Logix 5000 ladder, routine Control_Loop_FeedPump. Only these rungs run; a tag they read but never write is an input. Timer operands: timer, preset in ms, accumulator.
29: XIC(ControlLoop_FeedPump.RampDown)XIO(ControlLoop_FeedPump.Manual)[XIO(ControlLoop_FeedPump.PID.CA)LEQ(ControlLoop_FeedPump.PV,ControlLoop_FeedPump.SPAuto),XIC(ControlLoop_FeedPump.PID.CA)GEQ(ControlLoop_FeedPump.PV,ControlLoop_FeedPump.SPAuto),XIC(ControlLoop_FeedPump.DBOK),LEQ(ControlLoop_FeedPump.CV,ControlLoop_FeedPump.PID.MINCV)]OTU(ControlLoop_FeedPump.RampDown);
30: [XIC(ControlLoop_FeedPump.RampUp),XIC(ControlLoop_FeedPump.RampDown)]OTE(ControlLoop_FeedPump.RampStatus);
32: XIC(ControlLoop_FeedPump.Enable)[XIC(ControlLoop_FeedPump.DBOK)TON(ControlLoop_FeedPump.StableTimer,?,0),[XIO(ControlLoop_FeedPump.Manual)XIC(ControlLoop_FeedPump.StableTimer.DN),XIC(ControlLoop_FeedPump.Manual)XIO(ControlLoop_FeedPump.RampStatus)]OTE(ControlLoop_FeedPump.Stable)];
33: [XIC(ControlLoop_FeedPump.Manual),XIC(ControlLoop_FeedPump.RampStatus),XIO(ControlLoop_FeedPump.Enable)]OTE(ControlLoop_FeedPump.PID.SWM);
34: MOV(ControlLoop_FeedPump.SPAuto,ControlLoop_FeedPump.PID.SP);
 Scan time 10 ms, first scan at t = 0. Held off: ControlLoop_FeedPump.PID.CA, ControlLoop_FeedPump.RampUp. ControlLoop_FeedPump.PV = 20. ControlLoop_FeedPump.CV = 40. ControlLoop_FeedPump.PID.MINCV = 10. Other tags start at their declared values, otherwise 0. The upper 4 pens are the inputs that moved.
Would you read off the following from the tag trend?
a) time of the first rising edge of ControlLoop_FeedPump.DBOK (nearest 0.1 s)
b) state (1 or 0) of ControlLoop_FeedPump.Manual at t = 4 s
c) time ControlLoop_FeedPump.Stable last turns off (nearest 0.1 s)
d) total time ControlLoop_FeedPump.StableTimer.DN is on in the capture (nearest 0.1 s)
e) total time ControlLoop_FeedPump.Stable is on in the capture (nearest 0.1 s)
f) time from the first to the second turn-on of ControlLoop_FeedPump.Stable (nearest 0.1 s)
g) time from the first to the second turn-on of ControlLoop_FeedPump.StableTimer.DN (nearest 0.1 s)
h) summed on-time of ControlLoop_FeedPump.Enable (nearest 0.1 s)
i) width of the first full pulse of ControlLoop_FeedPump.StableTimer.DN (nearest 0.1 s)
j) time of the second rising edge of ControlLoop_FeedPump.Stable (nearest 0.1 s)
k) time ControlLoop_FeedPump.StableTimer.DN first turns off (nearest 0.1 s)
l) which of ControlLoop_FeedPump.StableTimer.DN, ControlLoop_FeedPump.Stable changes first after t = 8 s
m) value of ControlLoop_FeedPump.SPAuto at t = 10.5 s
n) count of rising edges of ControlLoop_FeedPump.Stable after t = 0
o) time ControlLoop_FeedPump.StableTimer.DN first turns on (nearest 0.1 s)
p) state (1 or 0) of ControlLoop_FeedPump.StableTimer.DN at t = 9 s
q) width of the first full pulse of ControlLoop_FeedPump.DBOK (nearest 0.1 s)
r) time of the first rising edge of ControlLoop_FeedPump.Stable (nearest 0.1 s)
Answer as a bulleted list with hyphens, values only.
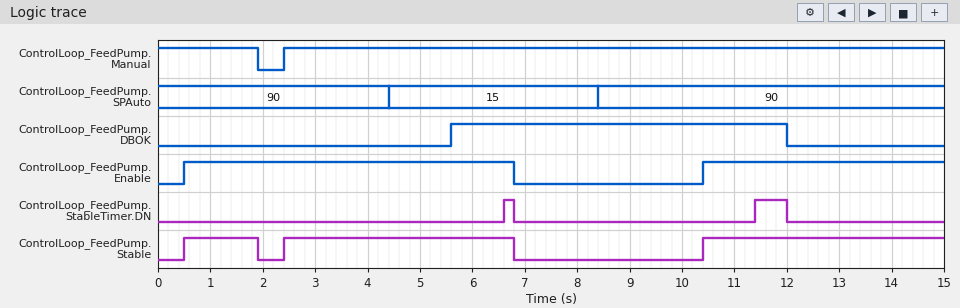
- 5.6 s
- 1
- 6.8 s
- 0.8 s
- 10.4 s
- 1.9 s
- 4.8 s
- 10.9 s
- 0.2 s
- 2.4 s
- 6.8 s
- ControlLoop_FeedPump.Stable
- 90
- 3
- 6.6 s
- 0
- 6.4 s
- 0.5 s
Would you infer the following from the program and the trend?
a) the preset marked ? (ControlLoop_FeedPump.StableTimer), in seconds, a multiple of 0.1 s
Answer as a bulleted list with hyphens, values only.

- 1.0 s
